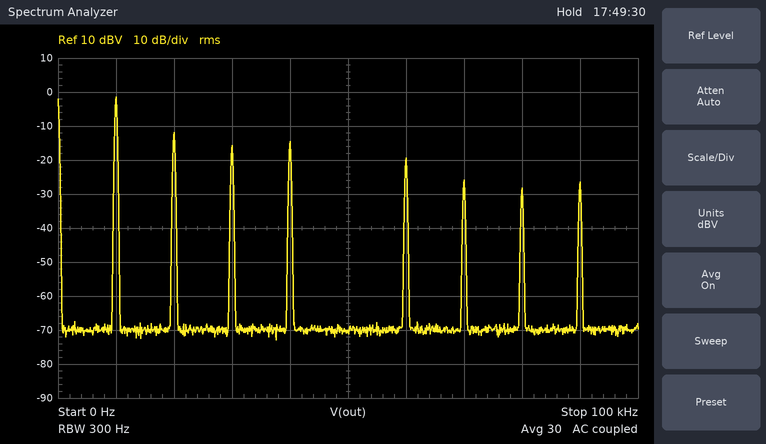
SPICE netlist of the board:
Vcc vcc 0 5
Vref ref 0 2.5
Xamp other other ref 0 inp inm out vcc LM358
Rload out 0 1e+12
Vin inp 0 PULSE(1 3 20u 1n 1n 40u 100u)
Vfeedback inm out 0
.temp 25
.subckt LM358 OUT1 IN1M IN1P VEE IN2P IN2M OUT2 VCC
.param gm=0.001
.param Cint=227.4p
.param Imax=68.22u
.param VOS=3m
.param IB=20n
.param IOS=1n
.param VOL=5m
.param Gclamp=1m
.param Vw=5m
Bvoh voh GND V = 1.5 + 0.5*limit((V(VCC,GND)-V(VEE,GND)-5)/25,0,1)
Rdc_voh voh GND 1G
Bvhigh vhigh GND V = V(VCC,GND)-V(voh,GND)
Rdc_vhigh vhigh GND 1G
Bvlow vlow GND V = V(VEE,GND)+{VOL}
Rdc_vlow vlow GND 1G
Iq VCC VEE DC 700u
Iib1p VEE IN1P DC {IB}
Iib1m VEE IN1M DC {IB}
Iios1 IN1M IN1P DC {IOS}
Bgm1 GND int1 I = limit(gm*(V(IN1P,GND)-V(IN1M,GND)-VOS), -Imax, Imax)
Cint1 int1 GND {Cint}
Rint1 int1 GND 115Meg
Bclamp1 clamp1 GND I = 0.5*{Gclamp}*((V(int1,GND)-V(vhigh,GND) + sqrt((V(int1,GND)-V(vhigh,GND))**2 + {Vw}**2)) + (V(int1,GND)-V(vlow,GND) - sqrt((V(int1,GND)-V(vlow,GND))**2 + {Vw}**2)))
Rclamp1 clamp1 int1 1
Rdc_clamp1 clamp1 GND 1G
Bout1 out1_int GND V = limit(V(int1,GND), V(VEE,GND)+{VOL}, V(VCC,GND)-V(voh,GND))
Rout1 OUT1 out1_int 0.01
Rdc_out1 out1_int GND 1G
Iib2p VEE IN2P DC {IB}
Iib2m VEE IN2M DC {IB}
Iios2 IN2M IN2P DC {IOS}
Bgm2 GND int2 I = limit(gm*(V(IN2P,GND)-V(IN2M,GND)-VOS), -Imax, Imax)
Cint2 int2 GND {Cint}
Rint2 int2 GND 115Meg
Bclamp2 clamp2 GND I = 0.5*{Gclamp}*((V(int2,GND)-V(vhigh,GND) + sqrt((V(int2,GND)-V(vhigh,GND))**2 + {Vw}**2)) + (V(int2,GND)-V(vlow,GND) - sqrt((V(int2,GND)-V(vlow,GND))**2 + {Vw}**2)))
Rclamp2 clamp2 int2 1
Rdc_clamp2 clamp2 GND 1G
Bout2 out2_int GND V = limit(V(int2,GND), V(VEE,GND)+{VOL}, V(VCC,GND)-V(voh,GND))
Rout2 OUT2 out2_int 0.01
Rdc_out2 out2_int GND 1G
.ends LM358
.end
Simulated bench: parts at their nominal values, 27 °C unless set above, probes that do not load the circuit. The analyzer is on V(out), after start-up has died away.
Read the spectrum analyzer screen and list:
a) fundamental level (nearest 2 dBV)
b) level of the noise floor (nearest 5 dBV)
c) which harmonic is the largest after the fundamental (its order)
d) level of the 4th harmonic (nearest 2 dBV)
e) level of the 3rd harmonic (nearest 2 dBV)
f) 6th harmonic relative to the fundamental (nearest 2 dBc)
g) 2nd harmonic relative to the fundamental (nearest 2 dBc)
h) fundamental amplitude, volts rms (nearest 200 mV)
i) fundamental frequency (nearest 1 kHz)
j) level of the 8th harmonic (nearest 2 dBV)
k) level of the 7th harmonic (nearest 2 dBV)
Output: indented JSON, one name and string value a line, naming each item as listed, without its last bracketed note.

{
  "fundamental level": "-2 dBV",
  "level of the noise floor": "-70 dBV",
  "which harmonic is the largest after the fundamental": "2",
  "level of the 4th harmonic": "-14 dBV",
  "level of the 3rd harmonic": "-16 dBV",
  "6th harmonic relative to the fundamental": "-18 dBc",
  "2nd harmonic relative to the fundamental": "-10 dBc",
  "fundamental amplitude, volts rms": "800 mV",
  "fundamental frequency": "10 kHz",
  "level of the 8th harmonic": "-28 dBV",
  "level of the 7th harmonic": "-26 dBV"
}
